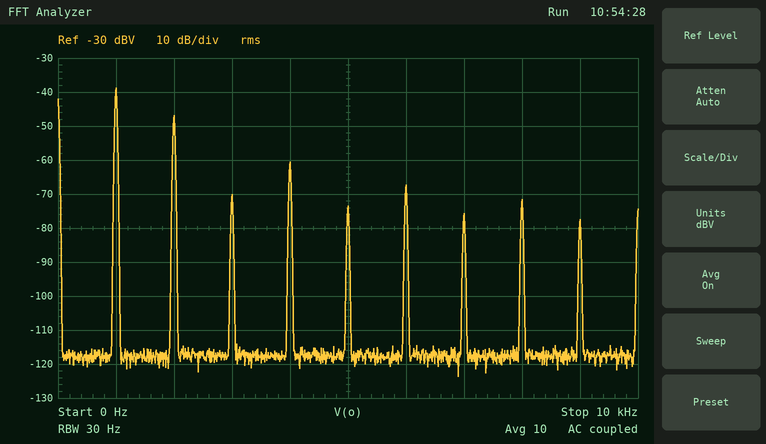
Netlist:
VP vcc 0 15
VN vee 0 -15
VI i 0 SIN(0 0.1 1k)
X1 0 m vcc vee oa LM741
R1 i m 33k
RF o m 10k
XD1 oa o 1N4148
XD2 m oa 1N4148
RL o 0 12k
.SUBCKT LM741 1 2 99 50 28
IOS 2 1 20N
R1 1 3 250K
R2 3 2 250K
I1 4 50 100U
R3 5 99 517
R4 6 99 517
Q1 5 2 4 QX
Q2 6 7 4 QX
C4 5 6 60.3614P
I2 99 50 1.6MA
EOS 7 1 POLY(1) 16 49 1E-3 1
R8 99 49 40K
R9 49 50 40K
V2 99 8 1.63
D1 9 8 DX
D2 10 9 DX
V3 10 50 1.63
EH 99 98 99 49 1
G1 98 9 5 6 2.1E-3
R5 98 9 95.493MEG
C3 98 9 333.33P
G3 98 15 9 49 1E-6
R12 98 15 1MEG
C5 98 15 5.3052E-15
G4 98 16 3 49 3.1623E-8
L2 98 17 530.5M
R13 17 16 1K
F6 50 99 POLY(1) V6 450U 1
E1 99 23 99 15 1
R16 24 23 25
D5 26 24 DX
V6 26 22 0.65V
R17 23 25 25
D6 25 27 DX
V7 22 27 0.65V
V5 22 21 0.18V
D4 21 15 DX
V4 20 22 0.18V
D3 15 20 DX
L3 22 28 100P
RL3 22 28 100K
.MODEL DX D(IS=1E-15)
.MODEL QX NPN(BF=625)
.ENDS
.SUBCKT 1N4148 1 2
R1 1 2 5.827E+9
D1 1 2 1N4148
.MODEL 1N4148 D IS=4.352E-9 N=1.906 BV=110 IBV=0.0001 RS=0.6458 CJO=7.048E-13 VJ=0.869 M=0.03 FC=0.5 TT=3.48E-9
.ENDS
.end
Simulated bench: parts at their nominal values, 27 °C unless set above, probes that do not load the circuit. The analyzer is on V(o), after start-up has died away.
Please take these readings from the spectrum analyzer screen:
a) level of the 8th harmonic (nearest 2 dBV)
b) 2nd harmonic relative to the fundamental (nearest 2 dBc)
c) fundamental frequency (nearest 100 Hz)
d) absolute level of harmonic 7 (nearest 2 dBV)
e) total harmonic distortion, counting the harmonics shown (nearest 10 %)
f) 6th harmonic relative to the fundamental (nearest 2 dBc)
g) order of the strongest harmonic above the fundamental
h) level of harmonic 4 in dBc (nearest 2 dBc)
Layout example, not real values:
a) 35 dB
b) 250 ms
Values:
a) -72 dBV
b) -8 dBc
c) 1.0 kHz
d) -76 dBV
e) 40 %
f) -28 dBc
g) 2
h) -22 dBc
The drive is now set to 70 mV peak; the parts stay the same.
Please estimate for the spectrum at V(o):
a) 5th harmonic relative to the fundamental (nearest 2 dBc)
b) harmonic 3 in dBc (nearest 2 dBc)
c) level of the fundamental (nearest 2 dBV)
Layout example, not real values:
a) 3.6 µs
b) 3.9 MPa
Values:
a) -32 dBc
b) -28 dBc
c) -42 dBV
